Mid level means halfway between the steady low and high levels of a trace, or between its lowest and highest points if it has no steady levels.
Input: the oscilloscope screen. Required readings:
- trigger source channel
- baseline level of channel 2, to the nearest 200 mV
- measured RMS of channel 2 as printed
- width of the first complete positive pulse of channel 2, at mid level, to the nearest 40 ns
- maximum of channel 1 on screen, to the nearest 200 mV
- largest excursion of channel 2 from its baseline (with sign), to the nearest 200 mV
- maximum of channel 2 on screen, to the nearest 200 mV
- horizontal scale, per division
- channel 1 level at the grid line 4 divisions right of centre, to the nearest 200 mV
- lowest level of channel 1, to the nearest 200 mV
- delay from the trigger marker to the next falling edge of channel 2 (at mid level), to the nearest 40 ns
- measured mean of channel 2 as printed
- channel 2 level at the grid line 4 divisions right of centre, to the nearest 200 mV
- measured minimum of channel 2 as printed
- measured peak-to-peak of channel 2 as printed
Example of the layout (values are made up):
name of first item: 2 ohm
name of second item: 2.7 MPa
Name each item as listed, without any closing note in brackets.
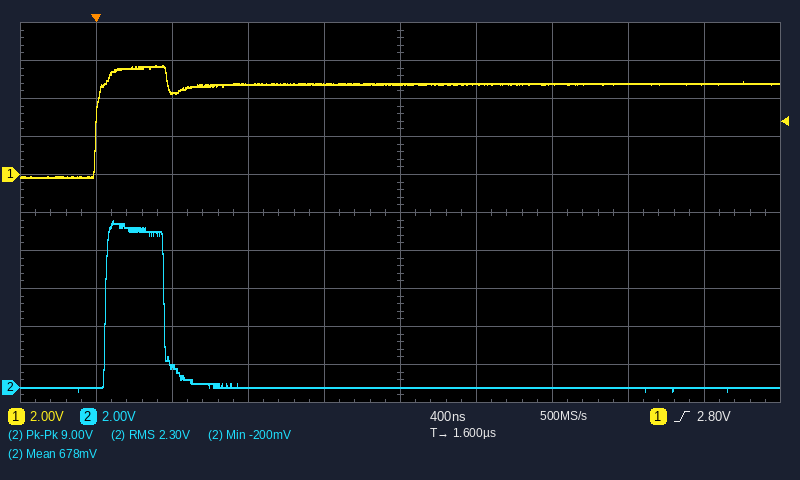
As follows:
trigger source channel: channel 1
baseline level of channel 2, to the nearest 200 mV: 0.0 V
measured RMS of channel 2 as printed: 2.30 V
width of the first complete positive pulse of channel 2, at mid level, to the nearest 40 ns: 320 ns
maximum of channel 1 on screen, to the nearest 200 mV: 5.8 V
largest excursion of channel 2 from its baseline (with sign), to the nearest 200 mV: +8.8 V
maximum of channel 2 on screen, to the nearest 200 mV: 8.8 V
horizontal scale, per division: 400 ns
channel 1 level at the grid line 4 divisions right of centre, to the nearest 200 mV: 4.8 V
lowest level of channel 1, to the nearest 200 mV: -200 mV
delay from the trigger marker to the next falling edge of channel 2 (at mid level), to the nearest 40 ns: 360 ns
measured mean of channel 2 as printed: 678 mV
channel 2 level at the grid line 4 divisions right of centre, to the nearest 200 mV: 0.0 V
measured minimum of channel 2 as printed: -200 mV
measured peak-to-peak of channel 2 as printed: 9.00 V
